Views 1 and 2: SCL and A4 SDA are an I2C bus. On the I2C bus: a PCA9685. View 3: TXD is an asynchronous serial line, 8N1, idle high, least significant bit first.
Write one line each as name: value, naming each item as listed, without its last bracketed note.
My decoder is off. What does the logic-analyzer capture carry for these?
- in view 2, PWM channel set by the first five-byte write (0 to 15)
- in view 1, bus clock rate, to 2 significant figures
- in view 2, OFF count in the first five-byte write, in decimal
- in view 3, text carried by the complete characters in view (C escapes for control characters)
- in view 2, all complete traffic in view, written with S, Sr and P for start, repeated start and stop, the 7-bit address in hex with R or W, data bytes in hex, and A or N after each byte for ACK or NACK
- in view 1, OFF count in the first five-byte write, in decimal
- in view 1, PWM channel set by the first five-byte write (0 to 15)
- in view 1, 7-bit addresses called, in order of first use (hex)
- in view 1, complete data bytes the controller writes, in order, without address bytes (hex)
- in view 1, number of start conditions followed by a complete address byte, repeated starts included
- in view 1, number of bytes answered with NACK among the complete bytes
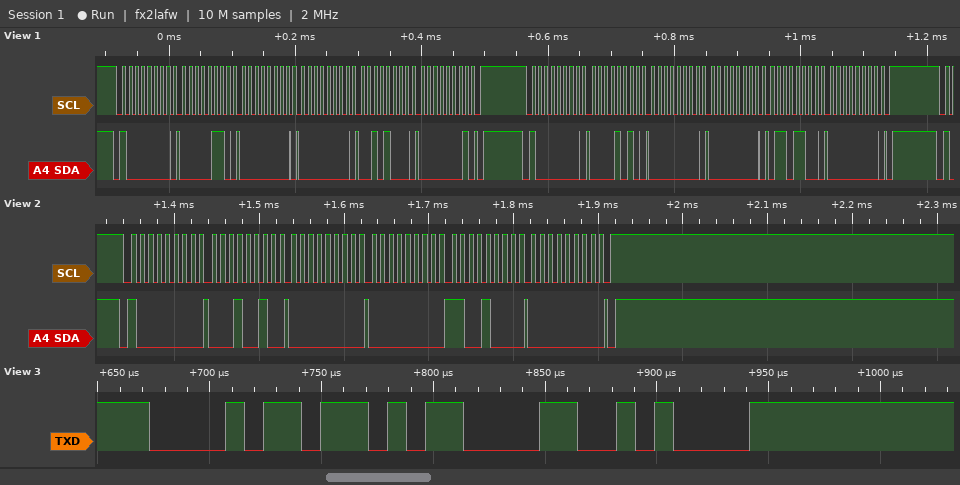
in view 2, PWM channel set by the first five-byte write: 3
in view 1, bus clock rate, to 2 significant figures: 100 kHz
in view 2, OFF count in the first five-byte write, in decimal: 200
in view 3, text carried by the complete characters in view: "h\r\n"
in view 2, all complete traffic in view, written with S, Sr and P for start, repeated start and stop, the 7-bit address in hex with R or W, data bytes in hex, and A or N after each byte for ACK or NACK: S 40W A 12 A 00 A 00 A C8 A 00 A P
in view 1, OFF count in the first five-byte write, in decimal: 296
in view 1, PWM channel set by the first five-byte write: 0
in view 1, 7-bit addresses called, in order of first use: 0x40
in view 1, complete data bytes the controller writes, in order, without address bytes: 06 00 00 28 01 0A 00 00 6C 00
in view 1, number of start conditions followed by a complete address byte, repeated starts included: 2
in view 1, number of bytes answered with NACK among the complete bytes: 0
